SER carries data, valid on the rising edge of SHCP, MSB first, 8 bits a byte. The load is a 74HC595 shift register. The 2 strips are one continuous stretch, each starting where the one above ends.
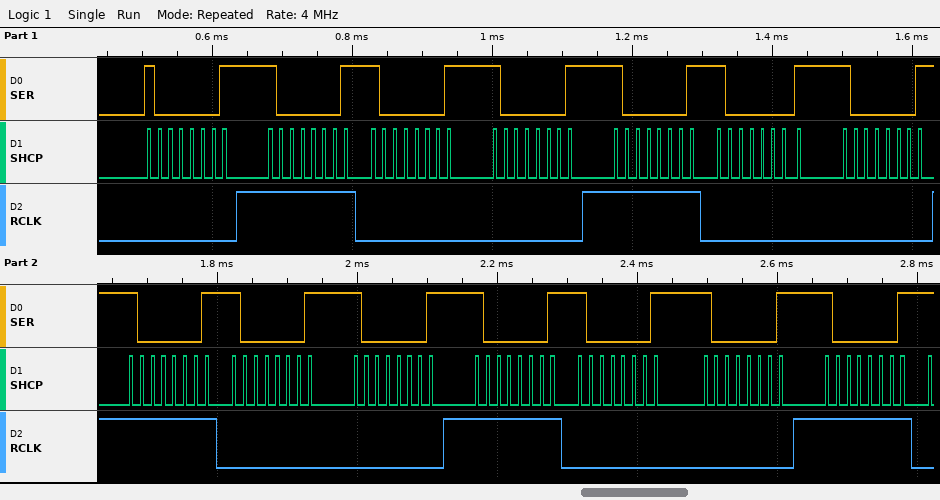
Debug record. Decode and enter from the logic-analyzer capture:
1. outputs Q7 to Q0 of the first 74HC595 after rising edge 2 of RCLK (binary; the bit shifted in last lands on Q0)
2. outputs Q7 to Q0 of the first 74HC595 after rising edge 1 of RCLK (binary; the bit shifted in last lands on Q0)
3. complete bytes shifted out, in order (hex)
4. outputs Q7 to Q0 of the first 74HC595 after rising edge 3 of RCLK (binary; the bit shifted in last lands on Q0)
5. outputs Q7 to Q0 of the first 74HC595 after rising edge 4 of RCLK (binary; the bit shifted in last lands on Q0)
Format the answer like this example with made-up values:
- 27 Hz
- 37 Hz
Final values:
- 10000001
- 10000001
- 81 81 81 81 81 81 81 81 81 81 81 81 81 81
- 10000001
- 10000001
